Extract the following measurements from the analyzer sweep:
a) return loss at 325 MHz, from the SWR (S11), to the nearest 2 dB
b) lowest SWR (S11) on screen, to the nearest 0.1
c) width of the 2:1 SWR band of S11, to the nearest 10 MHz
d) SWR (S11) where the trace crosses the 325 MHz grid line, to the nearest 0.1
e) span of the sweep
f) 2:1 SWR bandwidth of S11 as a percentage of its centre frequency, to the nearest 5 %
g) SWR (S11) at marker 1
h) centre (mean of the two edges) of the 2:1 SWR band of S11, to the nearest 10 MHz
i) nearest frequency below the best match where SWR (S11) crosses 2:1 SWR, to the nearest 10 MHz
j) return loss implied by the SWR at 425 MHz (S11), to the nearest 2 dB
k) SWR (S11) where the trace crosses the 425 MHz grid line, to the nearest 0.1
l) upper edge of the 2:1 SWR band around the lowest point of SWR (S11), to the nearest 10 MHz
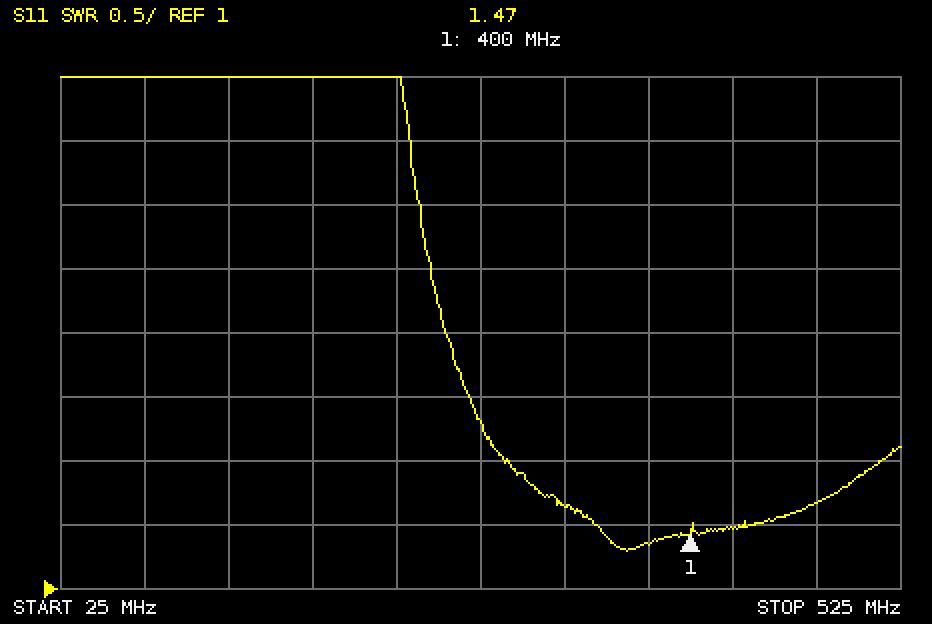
12 dB
1.3
220 MHz
1.6
500 MHz
55 %
1.47
400 MHz
290 MHz
14 dB
1.5
510 MHz
